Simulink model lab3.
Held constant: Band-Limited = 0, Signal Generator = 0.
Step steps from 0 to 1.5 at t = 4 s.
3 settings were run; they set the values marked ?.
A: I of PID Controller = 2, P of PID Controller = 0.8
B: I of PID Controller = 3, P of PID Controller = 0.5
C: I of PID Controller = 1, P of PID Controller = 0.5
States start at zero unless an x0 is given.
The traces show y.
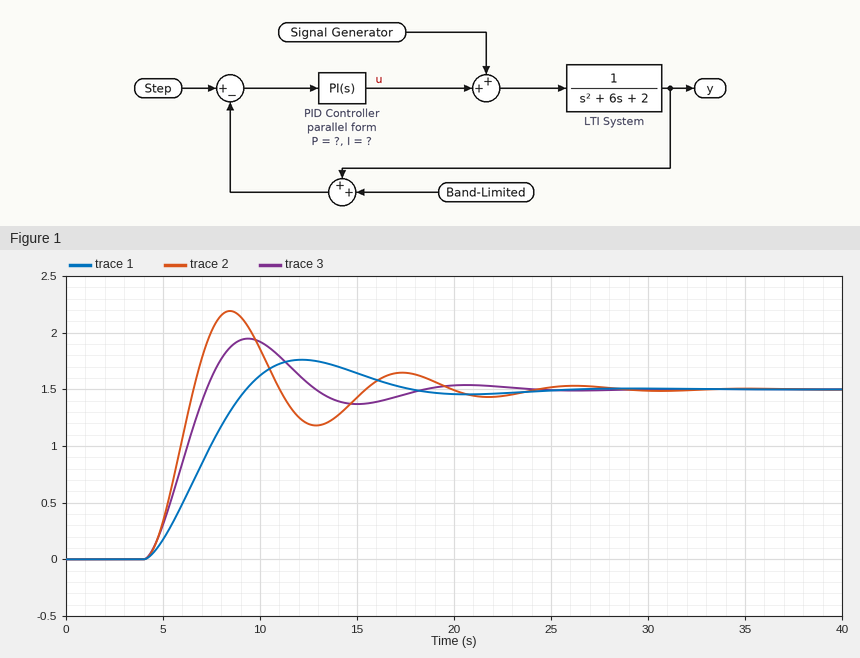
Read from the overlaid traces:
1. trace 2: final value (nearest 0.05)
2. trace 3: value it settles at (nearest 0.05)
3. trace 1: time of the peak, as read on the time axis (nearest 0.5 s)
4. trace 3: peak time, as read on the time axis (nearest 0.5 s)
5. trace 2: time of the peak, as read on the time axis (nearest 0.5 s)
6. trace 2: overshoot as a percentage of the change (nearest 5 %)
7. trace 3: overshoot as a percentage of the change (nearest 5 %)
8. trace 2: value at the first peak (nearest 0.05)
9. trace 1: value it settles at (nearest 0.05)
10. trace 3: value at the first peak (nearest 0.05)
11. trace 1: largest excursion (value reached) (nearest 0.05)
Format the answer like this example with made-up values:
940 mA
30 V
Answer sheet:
1.50
1.50
12.0 s
9.5 s
8.5 s
45 %
30 %
2.20
1.50
1.95
1.75
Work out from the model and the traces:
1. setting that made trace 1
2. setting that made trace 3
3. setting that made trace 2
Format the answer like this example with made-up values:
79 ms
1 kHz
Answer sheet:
C
A
B
